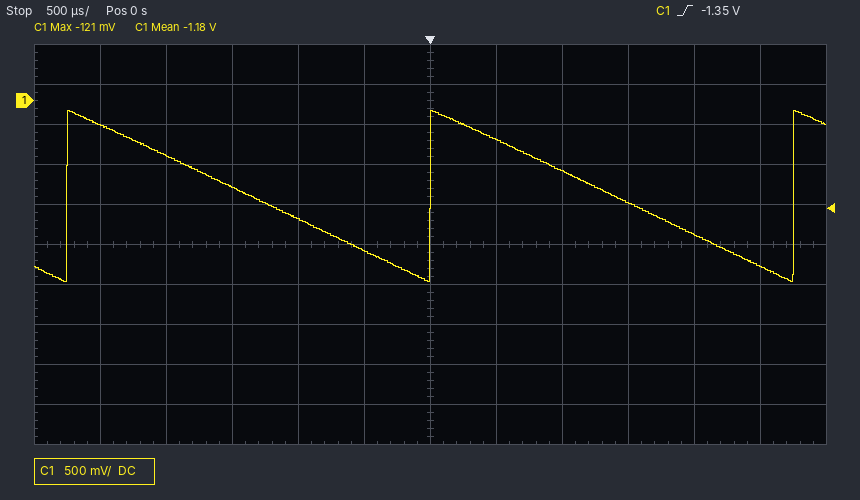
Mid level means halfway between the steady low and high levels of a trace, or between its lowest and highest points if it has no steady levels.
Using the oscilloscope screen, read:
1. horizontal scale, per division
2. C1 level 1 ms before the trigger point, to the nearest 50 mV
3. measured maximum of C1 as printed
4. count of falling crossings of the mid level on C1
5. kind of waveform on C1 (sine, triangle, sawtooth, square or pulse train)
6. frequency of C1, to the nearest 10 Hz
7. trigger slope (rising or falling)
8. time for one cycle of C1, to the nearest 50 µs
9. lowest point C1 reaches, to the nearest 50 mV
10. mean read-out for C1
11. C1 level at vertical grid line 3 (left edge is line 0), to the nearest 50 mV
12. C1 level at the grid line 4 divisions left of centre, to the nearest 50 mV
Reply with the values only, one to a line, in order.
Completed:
500 µs
-1.50 V
-121 mV
2
sawtooth
360 Hz
rising
2.75 ms
-2.25 V
-1.18 V
-1.10 V
-700 mV
